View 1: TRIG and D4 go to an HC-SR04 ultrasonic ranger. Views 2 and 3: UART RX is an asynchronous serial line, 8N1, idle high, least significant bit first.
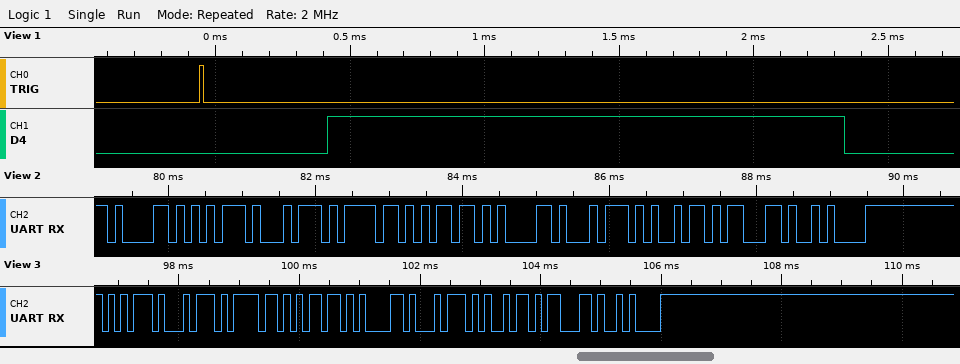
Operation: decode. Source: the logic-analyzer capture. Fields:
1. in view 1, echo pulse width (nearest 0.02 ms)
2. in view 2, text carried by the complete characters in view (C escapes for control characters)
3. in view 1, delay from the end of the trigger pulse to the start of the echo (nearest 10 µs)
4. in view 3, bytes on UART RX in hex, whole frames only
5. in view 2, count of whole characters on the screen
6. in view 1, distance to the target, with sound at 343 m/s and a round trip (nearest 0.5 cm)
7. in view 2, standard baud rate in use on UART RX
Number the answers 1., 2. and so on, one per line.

1. 1.92 ms
2. "automatic\n"
3. 460 µs
4. 0x75 0x74 0x6F 0x6D 0x61 0x74 0x69 0x63 0x0A
5. 10
6. 33 cm
7. 9600 baud
